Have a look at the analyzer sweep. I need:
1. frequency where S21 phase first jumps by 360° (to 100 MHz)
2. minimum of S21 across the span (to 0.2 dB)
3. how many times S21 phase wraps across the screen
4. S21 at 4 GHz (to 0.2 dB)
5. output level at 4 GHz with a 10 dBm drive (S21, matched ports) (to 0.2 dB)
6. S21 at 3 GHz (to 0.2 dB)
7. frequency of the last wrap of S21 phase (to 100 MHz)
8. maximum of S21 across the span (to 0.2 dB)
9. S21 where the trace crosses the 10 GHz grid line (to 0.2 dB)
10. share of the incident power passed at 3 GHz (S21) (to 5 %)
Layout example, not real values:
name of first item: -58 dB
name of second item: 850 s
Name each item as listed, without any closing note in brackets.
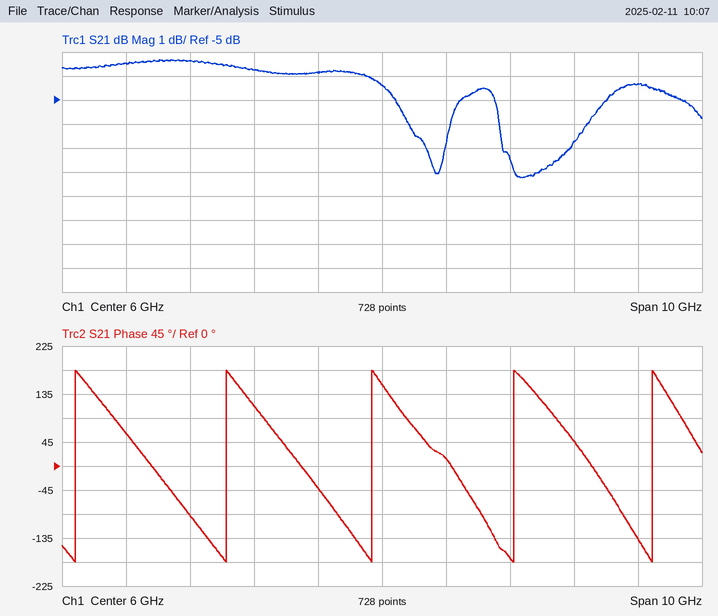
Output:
frequency where S21 phase first jumps by 360°: 1.2 GHz
minimum of S21 across the span: -8.2 dB
how many times S21 phase wraps across the screen: 5
S21 at 4 GHz: -3.8 dB
output level at 4 GHz with a 10 dBm drive (S21, matched ports): 6.2 dBm
S21 at 3 GHz: -3.4 dB
frequency of the last wrap of S21 phase: 10.2 GHz
maximum of S21 across the span: -3.4 dB
S21 where the trace crosses the 10 GHz grid line: -4.4 dB
share of the incident power passed at 3 GHz (S21): 45 %
